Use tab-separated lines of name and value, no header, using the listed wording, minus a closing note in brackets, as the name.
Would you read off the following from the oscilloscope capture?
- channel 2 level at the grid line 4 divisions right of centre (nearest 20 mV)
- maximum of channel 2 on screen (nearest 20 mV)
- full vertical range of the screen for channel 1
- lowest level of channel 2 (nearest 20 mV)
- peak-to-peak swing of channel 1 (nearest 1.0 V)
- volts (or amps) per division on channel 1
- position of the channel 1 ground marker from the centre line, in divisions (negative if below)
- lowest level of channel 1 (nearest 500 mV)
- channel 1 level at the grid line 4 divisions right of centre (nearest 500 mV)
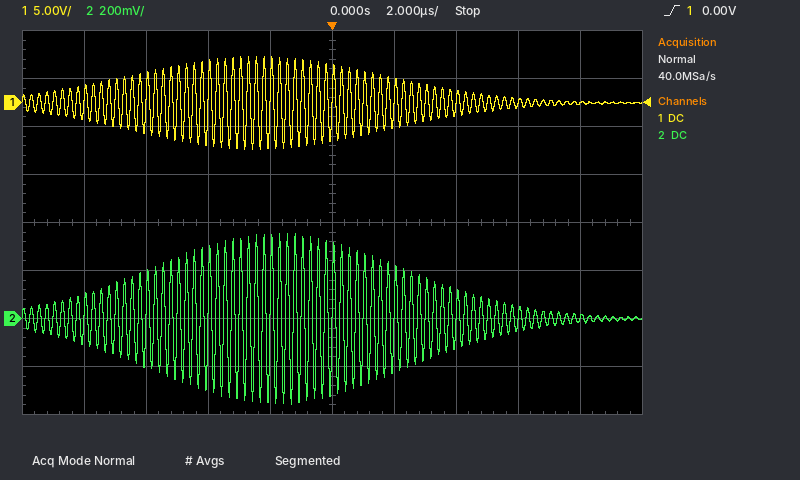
channel 2 level at the grid line 4 divisions right of centre	0 mV
maximum of channel 2 on screen	360 mV
full vertical range of the screen for channel 1	40 V
lowest level of channel 2	-360 mV
peak-to-peak swing of channel 1	10.0 V
volts (or amps) per division on channel 1	5 V
position of the channel 1 ground marker from the centre line, in divisions	+2.5 div
lowest level of channel 1	-5.0 V
channel 1 level at the grid line 4 divisions right of centre	0.0 V
